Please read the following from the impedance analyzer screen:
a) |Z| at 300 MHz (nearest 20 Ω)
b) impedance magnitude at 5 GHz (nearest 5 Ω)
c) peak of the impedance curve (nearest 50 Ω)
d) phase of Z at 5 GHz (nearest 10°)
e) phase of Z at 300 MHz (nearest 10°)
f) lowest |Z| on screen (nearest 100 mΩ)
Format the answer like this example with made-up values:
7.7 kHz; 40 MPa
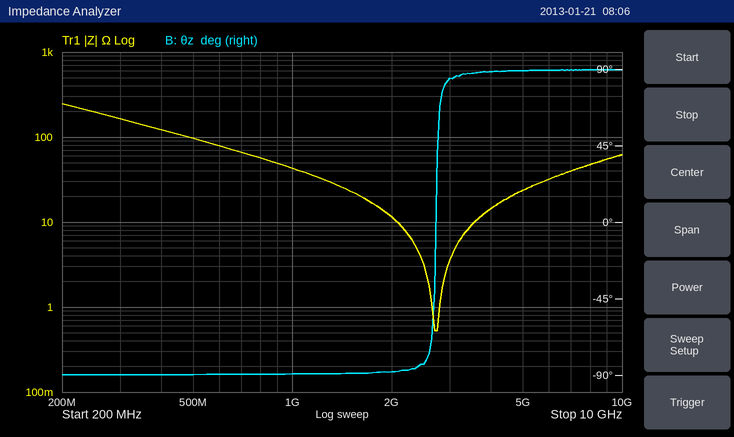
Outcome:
160 Ω; 25 Ω; 250 Ω; 90°; -90°; 500 mΩ
